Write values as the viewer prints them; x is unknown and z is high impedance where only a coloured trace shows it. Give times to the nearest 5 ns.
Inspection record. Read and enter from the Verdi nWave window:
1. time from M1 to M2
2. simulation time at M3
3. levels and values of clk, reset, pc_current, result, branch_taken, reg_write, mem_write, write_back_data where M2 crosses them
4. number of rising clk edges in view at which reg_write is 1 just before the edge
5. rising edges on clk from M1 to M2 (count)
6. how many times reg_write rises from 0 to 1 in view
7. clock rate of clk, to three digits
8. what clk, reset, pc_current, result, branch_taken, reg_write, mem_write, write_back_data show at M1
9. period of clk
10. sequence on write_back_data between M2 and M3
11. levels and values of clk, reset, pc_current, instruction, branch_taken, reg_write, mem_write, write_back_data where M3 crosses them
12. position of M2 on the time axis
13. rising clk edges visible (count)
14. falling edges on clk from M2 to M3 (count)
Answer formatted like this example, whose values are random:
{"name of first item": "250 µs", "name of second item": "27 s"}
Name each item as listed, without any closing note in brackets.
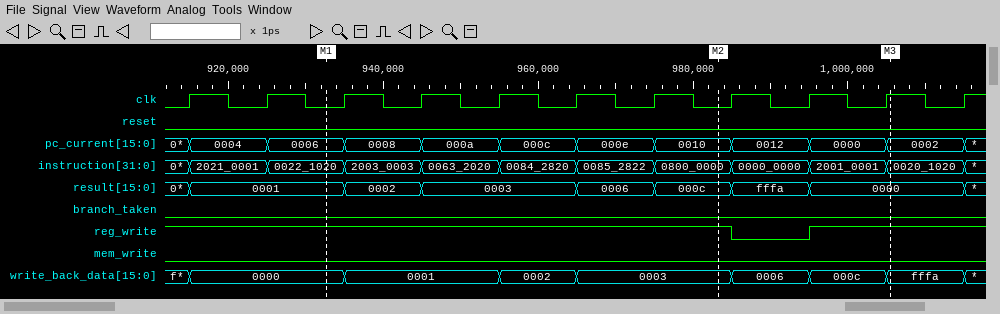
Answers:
{"time from M1 to M2": "50 ns", "simulation time at M3": "1005 ns", "levels and values of clk, reset, pc_current, result, branch_taken, reg_write, mem_write, write_back_data where M2 crosses them": "clk=0, reset=0, pc_current=0010, result=000c, branch_taken=0, reg_write=1, mem_write=0, write_back_data=0003", "number of rising clk edges in view at which reg_write is 1 just before the edge": "10", "rising edges on clk from M1 to M2": "5", "how many times reg_write rises from 0 to 1 in view": "1", "clock rate of clk, to three digits": "100 MHz", "what clk, reset, pc_current, result, branch_taken, reg_write, mem_write, write_back_data show at M1": "clk=0, reset=0, pc_current=0006, result=0001, branch_taken=0, reg_write=1, mem_write=0, write_back_data=0000", "period of clk": "10 ns", "sequence on write_back_data between M2 and M3": "0003, 0006, 000c, fffa", "levels and values of clk, reset, pc_current, instruction, branch_taken, reg_write, mem_write, write_back_data where M3 crosses them": "clk=1, reset=0, pc_current=0002, instruction=0020_1020, branch_taken=0, reg_write=1, mem_write=0, write_back_data=fffa", "position of M2 on the time axis": "985 ns", "rising clk edges visible": "11", "falling edges on clk from M2 to M3": "2"}
